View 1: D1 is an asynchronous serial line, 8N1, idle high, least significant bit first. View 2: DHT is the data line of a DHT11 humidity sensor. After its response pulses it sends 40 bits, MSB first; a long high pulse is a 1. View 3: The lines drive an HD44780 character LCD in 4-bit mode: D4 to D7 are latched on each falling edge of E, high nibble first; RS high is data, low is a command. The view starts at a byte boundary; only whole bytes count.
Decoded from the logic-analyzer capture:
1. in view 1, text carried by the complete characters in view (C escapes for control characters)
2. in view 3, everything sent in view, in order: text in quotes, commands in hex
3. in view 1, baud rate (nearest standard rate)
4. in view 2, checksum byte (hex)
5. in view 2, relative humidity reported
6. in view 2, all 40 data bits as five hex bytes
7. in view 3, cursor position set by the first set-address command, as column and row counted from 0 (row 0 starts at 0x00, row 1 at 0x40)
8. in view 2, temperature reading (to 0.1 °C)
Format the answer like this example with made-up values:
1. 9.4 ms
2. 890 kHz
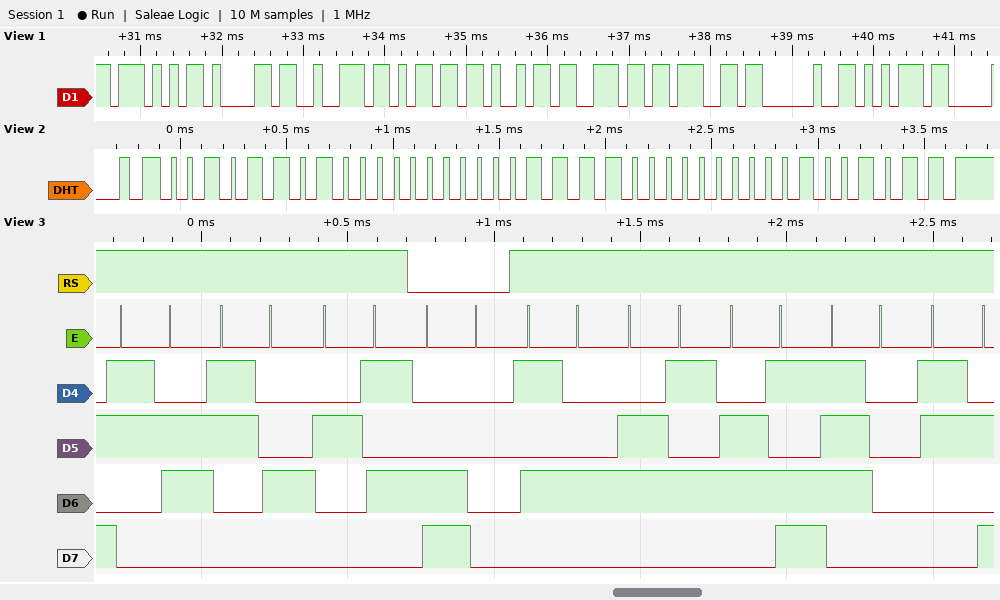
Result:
1. "Warming u"
2. "64%" 0xC0 "Temp:"
3. 9600 baud
4. 0x4B
5. 45 %
6. 2D 00 1E 00 4B
7. column 0, row 1
8. 30.0 °C
